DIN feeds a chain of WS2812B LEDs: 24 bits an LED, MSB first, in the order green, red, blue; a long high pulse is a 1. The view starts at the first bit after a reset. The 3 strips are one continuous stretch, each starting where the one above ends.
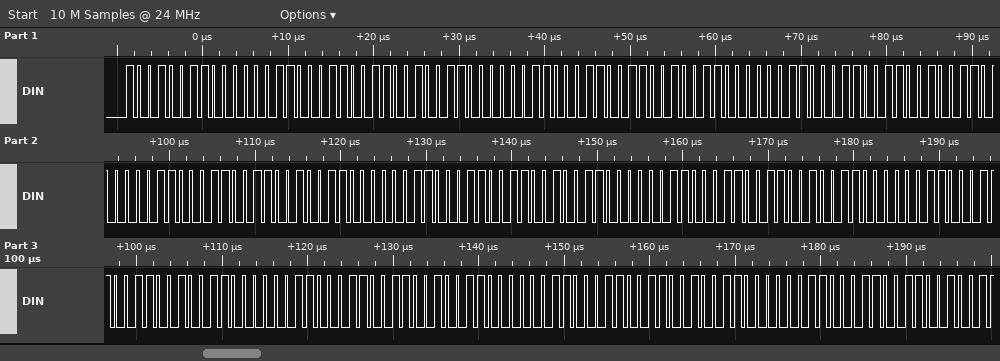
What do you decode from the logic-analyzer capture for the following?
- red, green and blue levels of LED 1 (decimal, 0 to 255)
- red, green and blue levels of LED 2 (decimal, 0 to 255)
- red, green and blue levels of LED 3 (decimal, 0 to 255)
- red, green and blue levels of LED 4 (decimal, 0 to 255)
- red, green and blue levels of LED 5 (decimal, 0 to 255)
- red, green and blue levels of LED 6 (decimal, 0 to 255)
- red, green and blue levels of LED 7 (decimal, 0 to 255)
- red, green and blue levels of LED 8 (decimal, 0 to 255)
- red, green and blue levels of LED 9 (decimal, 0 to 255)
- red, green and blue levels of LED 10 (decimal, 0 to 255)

3, 147, 25
3, 147, 25
3, 147, 25
3, 147, 25
3, 147, 25
3, 147, 25
3, 147, 25
3, 147, 25
3, 147, 25
3, 147, 25
